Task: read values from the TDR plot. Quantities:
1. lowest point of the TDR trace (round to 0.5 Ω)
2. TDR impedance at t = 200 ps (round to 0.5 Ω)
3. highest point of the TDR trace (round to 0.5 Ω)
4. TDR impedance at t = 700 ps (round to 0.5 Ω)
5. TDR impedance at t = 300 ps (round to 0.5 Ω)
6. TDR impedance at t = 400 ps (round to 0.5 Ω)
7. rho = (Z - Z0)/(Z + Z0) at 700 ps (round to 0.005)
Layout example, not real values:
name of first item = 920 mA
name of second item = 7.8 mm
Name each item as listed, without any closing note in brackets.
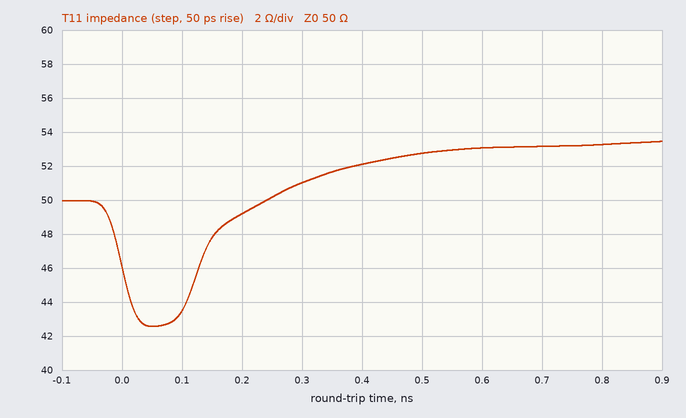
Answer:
lowest point of the TDR trace = 42.5 Ω
TDR impedance at t = 200 ps = 49.0 Ω
highest point of the TDR trace = 53.5 Ω
TDR impedance at t = 700 ps = 53.0 Ω
TDR impedance at t = 300 ps = 51.0 Ω
TDR impedance at t = 400 ps = 52.0 Ω
rho = (Z - Z0)/(Z + Z0) at 700 ps = +0.030
